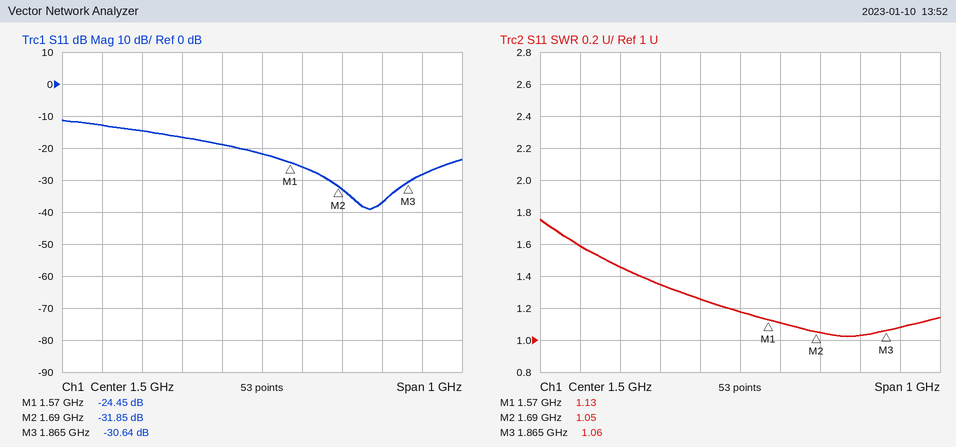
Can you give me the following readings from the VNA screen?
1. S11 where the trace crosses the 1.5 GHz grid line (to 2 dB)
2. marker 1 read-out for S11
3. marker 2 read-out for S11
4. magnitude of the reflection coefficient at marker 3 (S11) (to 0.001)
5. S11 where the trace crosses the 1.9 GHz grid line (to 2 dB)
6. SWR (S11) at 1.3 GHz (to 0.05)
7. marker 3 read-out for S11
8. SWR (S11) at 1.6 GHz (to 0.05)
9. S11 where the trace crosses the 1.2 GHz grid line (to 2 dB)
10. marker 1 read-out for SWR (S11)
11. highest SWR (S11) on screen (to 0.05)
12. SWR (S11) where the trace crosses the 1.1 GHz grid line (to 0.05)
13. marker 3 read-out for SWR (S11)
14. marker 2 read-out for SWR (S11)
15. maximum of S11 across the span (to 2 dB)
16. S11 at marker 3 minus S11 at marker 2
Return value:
-22 dB
-24.45 dB
-31.85 dB
0.029
-28 dB
1.35
-30.64 dB
1.10
-14 dB
1.13
1.75
1.60
1.06
1.05
-12 dB
1.21 dB
